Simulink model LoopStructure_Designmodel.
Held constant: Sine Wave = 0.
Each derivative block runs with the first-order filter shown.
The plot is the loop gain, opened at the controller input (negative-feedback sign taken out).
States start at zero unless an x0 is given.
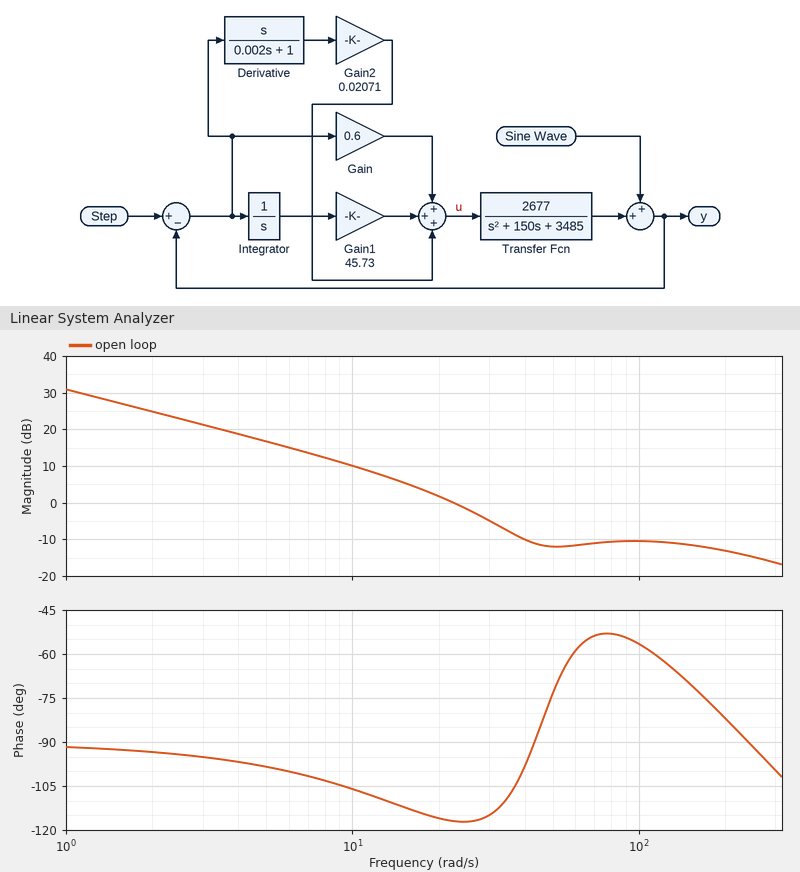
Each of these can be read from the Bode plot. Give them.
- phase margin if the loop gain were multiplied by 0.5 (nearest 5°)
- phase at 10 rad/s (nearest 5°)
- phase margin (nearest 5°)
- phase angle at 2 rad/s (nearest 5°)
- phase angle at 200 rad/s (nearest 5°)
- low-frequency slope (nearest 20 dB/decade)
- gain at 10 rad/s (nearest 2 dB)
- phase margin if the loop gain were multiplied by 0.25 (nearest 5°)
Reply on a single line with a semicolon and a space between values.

70°; -105°; 65°; -95°; -80°; -20 dB/decade; 10 dB; 75°
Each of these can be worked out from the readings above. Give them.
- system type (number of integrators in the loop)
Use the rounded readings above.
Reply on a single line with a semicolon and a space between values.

1
